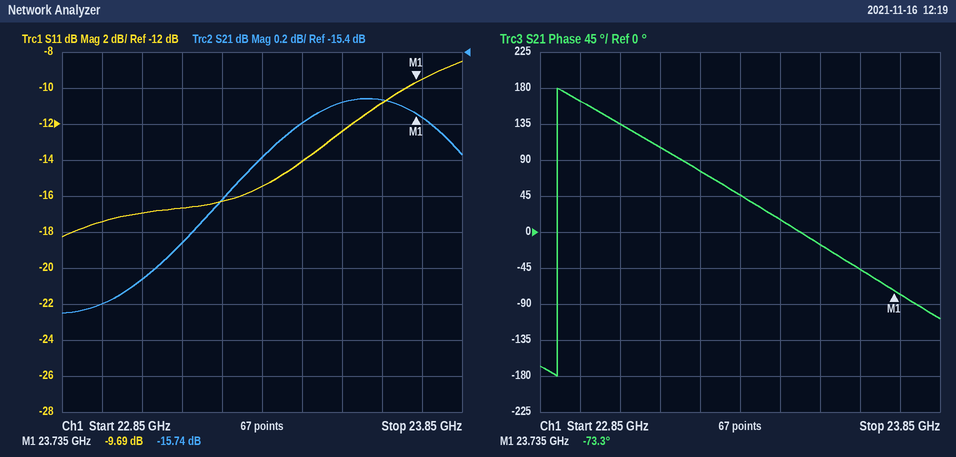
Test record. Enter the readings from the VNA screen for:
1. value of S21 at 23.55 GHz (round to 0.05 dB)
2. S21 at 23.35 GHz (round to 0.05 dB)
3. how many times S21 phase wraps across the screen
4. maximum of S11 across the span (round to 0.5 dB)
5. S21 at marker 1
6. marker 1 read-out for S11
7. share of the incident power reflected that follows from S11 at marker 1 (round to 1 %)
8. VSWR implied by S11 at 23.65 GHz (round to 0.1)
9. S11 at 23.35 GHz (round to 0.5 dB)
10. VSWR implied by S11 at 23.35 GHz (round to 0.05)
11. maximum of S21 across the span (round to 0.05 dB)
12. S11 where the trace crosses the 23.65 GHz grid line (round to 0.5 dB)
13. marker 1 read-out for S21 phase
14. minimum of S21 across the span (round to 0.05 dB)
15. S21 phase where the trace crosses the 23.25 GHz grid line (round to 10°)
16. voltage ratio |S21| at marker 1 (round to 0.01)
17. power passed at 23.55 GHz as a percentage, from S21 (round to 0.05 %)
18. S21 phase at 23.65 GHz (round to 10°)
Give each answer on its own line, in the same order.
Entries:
-15.70 dB
-16.00 dB
1
-8.5 dB
-15.74 dB
-9.69 dB
11 %
1.8
-15.5 dB
1.40
-15.65 dB
-11.0 dB
-73.3°
-16.85 dB
80°
0.16
2.70 %
-50°
